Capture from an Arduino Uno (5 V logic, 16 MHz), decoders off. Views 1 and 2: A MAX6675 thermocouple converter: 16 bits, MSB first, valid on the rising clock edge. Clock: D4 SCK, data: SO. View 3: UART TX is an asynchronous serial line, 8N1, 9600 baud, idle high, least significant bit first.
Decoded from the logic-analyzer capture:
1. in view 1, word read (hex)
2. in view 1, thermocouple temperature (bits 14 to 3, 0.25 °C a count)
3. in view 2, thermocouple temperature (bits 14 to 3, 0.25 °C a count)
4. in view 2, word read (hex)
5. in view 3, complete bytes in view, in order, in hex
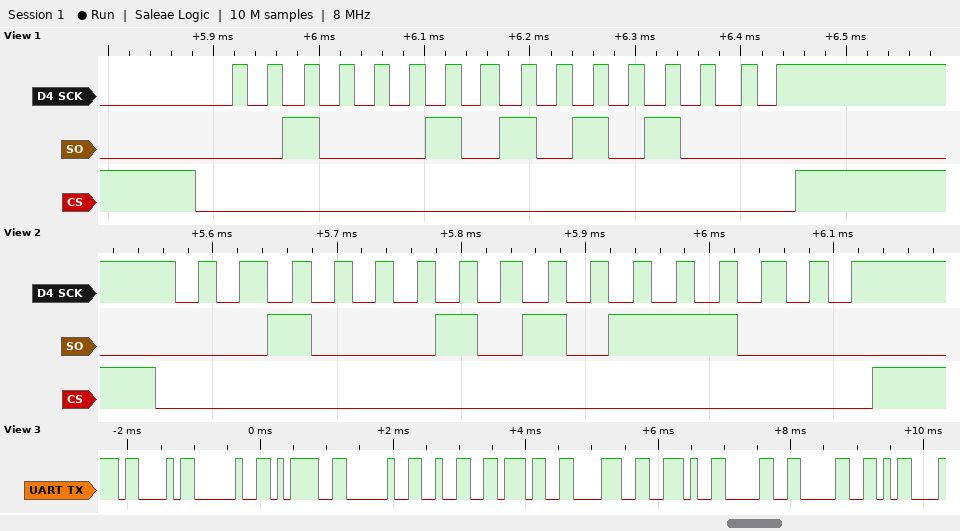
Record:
0x22A8
277.25 °C
277.75 °C
0x22B8
43 20 3D 20 32 37 38 2E 30 30 0D
